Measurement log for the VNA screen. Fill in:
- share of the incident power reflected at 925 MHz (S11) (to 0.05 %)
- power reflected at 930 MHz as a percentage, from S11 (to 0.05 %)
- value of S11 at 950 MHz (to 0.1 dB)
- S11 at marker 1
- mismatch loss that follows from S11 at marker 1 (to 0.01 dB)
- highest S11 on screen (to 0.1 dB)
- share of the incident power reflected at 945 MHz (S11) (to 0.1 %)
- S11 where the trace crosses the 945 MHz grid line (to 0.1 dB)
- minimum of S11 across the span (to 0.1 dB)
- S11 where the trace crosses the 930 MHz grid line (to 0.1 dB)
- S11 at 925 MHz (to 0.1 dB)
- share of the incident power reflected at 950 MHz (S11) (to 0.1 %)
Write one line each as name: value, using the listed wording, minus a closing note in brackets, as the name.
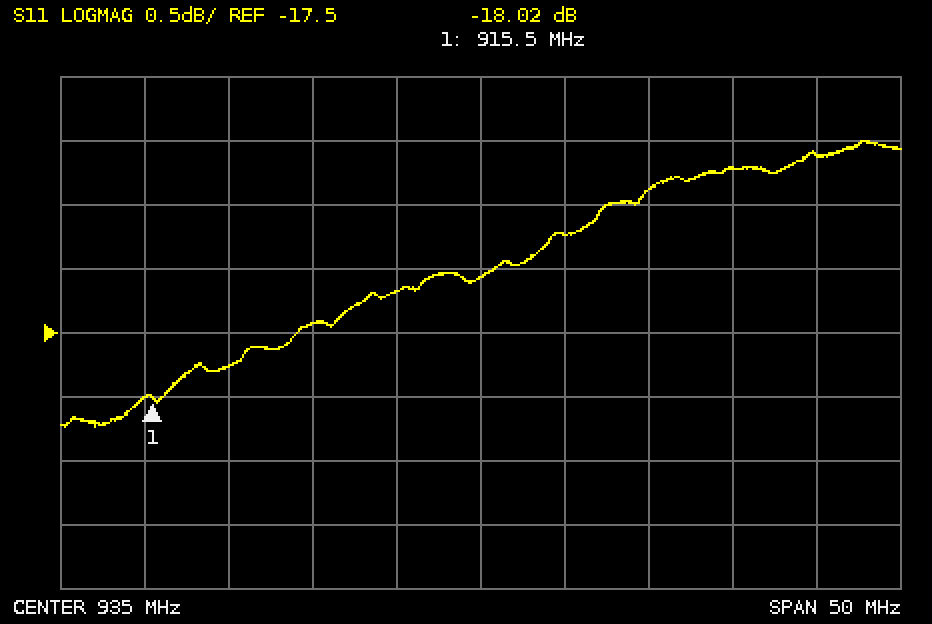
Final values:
share of the incident power reflected at 925 MHz (S11): 1.80 %
power reflected at 930 MHz as a percentage, from S11: 1.90 %
value of S11 at 950 MHz: -16.2 dB
S11 at marker 1: -18.02 dB
mismatch loss that follows from S11 at marker 1: 0.07 dB
highest S11 on screen: -16.0 dB
share of the incident power reflected at 945 MHz (S11): 2.3 %
S11 where the trace crosses the 945 MHz grid line: -16.4 dB
minimum of S11 across the span: -18.2 dB
S11 where the trace crosses the 930 MHz grid line: -17.2 dB
S11 at 925 MHz: -17.4 dB
share of the incident power reflected at 950 MHz (S11): 2.4 %
